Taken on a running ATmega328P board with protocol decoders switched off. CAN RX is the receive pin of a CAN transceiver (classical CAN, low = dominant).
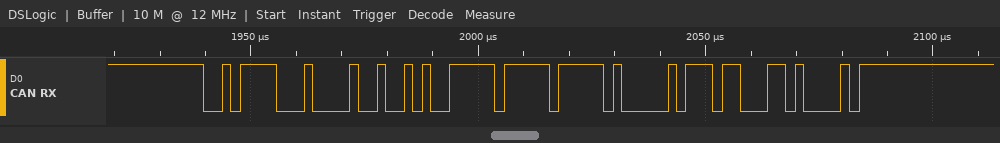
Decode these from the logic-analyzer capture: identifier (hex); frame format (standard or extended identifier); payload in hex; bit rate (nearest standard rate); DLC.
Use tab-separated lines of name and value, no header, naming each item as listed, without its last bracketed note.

identifier	0x2F1
frame format	standard
payload in hex	94 FF FF 03
bit rate	500 kbit/s
DLC	4
